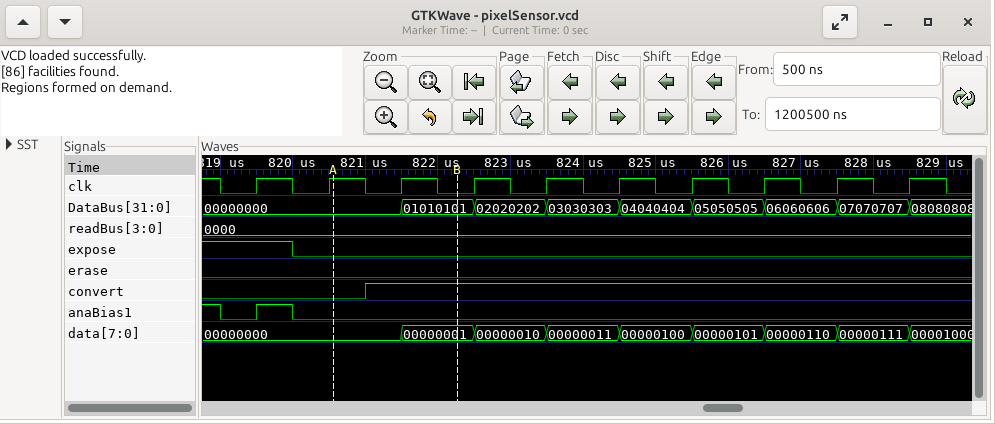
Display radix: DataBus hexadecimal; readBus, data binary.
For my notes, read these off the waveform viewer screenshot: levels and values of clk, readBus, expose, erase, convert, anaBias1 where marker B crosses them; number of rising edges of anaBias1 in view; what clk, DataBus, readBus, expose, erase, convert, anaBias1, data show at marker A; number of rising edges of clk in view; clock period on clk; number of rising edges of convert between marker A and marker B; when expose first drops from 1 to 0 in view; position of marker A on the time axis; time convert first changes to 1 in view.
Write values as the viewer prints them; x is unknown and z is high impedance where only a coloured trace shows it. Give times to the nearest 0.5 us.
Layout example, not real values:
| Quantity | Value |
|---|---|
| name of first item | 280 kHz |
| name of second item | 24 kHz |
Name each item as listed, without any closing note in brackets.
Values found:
| Quantity | Value |
|---|---|
| levels and values of clk, readBus, expose, erase, convert, anaBias1 where marker B crosses them | clk=0, readBus=0000, expose=0, erase=0, convert=1, anaBias1=0 |
| number of rising edges of anaBias1 in view | 1 |
| what clk, DataBus, readBus, expose, erase, convert, anaBias1, data show at marker A | clk=1, DataBus=00000000, readBus=0000, expose=0, erase=0, convert=0, anaBias1=0, data=00000000 |
| number of rising edges of clk in view | 10 |
| clock period on clk | 1 us |
| number of rising edges of convert between marker A and marker B | 1 |
| when expose first drops from 1 to 0 in view | 820 us |
| position of marker A on the time axis | 820.5 us |
| time convert first changes to 1 in view | 821 us |
